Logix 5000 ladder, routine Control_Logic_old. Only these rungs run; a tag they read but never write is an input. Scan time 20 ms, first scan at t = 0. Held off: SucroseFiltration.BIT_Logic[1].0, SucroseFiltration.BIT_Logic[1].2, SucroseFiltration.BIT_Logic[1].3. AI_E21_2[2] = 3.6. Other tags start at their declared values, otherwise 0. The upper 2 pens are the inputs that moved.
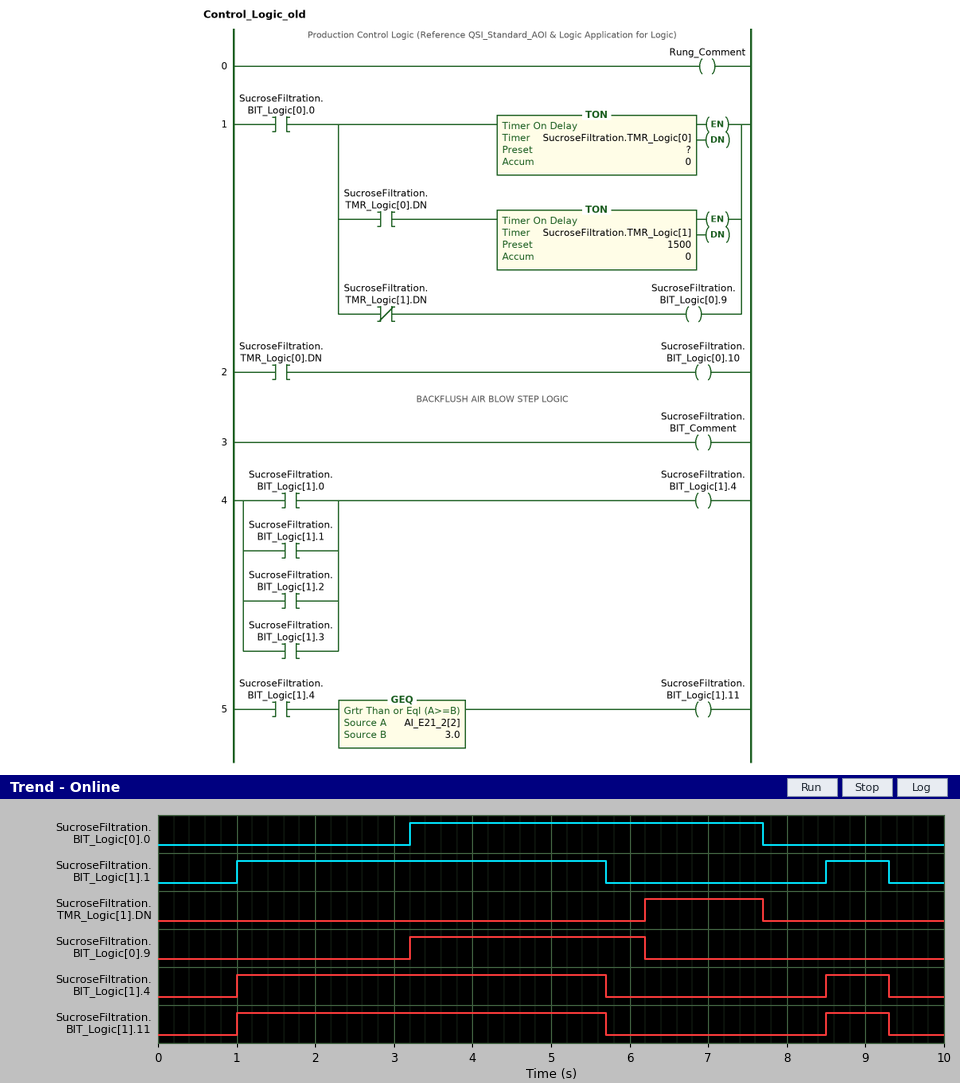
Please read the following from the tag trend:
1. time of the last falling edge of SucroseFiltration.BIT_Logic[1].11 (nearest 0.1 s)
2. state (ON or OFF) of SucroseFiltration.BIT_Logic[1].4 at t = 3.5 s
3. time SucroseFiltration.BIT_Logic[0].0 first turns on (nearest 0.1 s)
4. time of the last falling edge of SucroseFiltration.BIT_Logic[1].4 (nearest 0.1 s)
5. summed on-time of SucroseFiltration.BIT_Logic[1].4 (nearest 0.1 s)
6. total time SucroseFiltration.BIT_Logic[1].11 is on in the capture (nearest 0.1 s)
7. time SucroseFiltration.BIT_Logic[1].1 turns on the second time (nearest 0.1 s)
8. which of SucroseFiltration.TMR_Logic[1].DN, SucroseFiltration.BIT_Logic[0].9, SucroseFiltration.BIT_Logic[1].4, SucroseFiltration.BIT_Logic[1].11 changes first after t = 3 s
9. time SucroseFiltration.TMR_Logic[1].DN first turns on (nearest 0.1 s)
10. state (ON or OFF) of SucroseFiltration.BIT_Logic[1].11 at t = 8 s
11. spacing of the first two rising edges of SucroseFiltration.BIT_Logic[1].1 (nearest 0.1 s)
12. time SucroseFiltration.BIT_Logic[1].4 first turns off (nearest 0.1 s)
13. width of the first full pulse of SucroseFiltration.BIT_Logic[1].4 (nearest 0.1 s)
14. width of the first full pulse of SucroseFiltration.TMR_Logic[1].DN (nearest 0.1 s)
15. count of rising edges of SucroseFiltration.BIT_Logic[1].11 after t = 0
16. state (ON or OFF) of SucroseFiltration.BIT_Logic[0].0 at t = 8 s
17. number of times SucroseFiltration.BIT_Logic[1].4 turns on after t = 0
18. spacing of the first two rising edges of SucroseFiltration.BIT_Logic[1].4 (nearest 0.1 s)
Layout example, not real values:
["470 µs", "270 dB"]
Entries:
["9.3 s", "ON", "3.2 s", "9.3 s", "5.5 s", "5.5 s", "8.5 s", "SucroseFiltration.BIT_Logic[0].9", "6.2 s", "OFF", "7.5 s", "5.7 s", "4.7 s", "1.5 s", "2", "OFF", "2", "7.5 s"]
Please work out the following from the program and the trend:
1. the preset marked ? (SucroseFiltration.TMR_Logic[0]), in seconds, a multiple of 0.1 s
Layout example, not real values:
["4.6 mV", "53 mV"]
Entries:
["1.5 s"]
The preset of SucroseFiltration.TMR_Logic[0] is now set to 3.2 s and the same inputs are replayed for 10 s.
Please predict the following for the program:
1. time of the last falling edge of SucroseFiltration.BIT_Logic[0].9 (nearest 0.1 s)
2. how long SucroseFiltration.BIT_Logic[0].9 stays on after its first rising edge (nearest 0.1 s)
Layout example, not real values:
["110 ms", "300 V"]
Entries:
["7.7 s", "4.5 s"]
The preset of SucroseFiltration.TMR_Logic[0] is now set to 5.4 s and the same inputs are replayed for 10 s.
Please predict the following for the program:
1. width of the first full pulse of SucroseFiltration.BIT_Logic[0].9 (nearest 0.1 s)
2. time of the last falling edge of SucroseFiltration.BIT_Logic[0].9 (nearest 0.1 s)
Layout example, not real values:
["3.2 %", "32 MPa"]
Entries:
["4.5 s", "7.7 s"]
